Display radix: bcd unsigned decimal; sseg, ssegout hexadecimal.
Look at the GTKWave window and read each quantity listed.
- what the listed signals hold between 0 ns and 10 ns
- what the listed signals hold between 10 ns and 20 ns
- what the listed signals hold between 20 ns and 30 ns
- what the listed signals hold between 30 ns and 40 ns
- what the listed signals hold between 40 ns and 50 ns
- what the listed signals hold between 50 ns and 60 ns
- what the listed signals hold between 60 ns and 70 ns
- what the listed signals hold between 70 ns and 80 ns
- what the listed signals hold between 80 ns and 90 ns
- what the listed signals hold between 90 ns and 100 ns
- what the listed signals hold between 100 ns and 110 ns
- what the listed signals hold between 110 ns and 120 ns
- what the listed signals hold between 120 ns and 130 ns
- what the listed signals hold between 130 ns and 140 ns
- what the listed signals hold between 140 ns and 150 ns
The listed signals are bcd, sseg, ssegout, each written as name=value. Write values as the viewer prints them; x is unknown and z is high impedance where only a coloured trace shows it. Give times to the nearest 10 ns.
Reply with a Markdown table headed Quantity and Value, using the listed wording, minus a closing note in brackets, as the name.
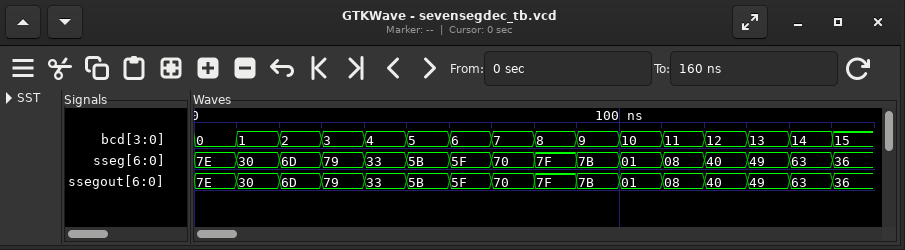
| Quantity | Value |
|---|---|
| what the listed signals hold between 0 ns and 10 ns | bcd=0, sseg=7E, ssegout=7E |
| what the listed signals hold between 10 ns and 20 ns | bcd=1, sseg=30, ssegout=30 |
| what the listed signals hold between 20 ns and 30 ns | bcd=2, sseg=6D, ssegout=6D |
| what the listed signals hold between 30 ns and 40 ns | bcd=3, sseg=79, ssegout=79 |
| what the listed signals hold between 40 ns and 50 ns | bcd=4, sseg=33, ssegout=33 |
| what the listed signals hold between 50 ns and 60 ns | bcd=5, sseg=5B, ssegout=5B |
| what the listed signals hold between 60 ns and 70 ns | bcd=6, sseg=5F, ssegout=5F |
| what the listed signals hold between 70 ns and 80 ns | bcd=7, sseg=70, ssegout=70 |
| what the listed signals hold between 80 ns and 90 ns | bcd=8, sseg=7F, ssegout=7F |
| what the listed signals hold between 90 ns and 100 ns | bcd=9, sseg=7B, ssegout=7B |
| what the listed signals hold between 100 ns and 110 ns | bcd=10, sseg=01, ssegout=01 |
| what the listed signals hold between 110 ns and 120 ns | bcd=11, sseg=08, ssegout=08 |
| what the listed signals hold between 120 ns and 130 ns | bcd=12, sseg=40, ssegout=40 |
| what the listed signals hold between 130 ns and 140 ns | bcd=13, sseg=49, ssegout=49 |
| what the listed signals hold between 140 ns and 150 ns | bcd=14, sseg=63, ssegout=63 |
